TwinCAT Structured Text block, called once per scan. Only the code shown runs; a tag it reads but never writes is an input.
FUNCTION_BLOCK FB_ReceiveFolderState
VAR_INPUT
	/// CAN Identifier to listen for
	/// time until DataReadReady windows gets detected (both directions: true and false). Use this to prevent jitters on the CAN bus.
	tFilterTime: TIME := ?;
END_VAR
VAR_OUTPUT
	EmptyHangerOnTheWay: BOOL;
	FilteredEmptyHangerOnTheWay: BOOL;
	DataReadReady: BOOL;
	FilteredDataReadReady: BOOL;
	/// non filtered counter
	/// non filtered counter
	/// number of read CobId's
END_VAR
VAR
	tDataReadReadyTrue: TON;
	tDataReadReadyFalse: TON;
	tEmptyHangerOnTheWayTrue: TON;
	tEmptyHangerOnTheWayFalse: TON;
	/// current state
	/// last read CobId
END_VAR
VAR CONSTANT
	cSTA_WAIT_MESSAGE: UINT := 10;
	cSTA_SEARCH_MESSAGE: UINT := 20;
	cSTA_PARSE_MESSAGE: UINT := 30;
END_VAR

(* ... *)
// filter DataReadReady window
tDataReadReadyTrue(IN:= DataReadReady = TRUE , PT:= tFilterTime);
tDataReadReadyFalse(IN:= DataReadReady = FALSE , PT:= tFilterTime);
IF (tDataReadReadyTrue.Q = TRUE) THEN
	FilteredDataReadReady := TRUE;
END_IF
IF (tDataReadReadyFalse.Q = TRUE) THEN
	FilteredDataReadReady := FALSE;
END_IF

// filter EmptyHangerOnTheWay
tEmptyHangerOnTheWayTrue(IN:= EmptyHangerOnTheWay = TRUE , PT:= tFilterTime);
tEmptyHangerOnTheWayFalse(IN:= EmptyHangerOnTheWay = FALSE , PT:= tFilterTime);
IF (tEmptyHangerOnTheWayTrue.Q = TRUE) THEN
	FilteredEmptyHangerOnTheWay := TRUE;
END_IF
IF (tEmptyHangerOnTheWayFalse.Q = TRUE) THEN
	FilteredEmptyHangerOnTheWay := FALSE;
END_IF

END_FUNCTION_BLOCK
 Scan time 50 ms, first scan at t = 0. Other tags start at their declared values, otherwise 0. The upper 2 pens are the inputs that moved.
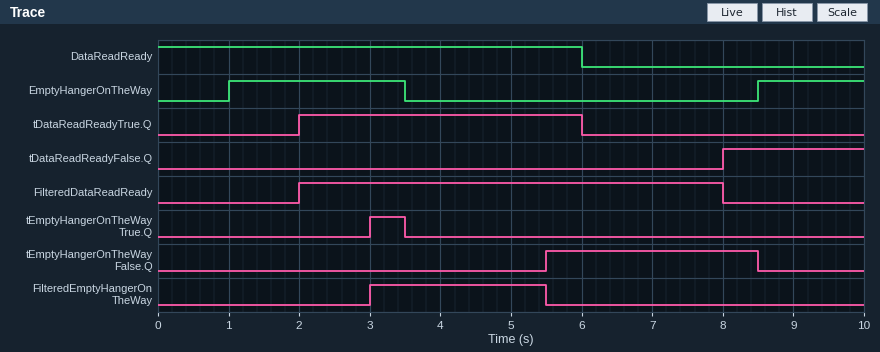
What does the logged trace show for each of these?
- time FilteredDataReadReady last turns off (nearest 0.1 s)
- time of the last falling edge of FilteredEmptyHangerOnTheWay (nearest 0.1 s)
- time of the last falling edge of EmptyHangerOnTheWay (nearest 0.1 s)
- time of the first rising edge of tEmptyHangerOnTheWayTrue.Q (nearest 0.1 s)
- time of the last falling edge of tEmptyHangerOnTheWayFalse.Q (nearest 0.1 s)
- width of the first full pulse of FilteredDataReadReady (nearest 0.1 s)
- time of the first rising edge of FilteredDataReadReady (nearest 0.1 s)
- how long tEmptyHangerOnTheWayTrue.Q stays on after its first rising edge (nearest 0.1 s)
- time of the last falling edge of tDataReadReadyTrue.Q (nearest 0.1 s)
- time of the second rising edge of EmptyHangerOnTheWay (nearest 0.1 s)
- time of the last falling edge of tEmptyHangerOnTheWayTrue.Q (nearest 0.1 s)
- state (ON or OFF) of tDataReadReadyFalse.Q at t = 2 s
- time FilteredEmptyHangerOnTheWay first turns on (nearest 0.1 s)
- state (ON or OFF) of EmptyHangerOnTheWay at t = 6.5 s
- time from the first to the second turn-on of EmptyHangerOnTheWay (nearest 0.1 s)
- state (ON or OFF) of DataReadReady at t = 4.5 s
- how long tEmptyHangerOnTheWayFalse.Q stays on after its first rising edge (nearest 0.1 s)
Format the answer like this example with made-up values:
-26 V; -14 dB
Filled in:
8.0 s; 5.5 s; 3.5 s; 3.0 s; 8.5 s; 6.0 s; 2.0 s; 0.5 s; 6.0 s; 8.5 s; 3.5 s; OFF; 3.0 s; OFF; 7.5 s; ON; 3.0 s
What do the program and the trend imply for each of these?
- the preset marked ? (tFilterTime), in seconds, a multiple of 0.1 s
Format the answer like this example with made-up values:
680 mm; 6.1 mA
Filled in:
2.0 s
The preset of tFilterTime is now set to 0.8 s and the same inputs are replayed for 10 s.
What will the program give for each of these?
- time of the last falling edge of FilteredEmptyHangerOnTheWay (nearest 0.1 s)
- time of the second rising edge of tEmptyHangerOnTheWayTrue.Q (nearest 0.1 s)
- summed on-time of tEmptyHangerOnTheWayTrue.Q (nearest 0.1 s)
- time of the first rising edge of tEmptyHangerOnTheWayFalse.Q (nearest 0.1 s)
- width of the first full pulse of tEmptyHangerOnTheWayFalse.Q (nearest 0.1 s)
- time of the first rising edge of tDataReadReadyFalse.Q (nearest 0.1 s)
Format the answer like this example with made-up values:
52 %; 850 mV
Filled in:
4.3 s; 9.3 s; 2.4 s; 0.8 s; 0.2 s; 6.8 s
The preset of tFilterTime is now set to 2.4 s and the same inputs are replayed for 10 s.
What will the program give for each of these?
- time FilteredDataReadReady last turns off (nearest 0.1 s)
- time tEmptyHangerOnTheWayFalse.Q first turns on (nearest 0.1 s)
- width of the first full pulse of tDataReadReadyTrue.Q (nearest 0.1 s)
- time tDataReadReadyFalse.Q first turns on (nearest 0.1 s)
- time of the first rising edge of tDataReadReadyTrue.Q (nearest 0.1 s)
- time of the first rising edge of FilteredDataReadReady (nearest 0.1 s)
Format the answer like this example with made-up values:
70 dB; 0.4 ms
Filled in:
8.4 s; 5.9 s; 3.6 s; 8.4 s; 2.4 s; 2.4 s
